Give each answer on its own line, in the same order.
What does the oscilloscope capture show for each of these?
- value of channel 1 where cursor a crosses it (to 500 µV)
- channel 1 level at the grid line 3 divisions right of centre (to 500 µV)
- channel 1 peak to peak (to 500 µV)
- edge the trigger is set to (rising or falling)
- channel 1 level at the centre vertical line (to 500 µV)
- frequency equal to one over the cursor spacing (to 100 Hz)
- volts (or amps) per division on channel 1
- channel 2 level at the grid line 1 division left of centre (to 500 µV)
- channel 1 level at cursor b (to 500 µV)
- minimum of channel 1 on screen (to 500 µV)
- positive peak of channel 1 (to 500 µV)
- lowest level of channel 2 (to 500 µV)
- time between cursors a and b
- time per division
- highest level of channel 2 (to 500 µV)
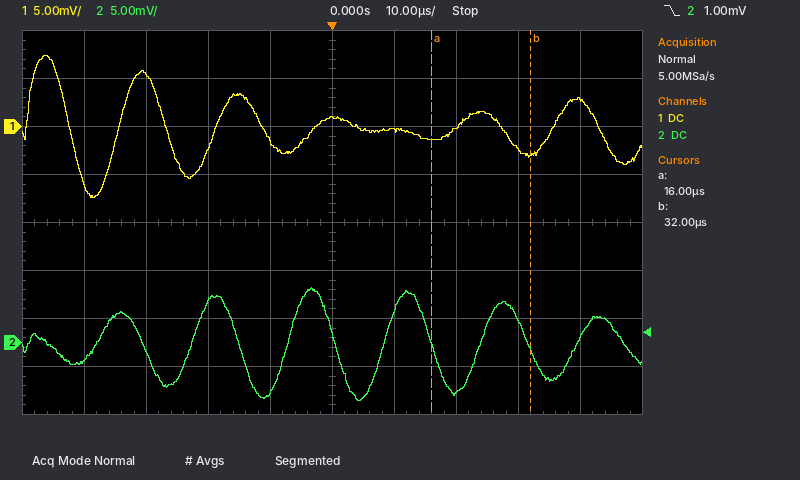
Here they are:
-1.5 mV
-2.5 mV
15.0 mV
falling
1.0 mV
62.5 kHz
5 mV
-5.0 mV
-3.0 mV
-7.5 mV
7.5 mV
-6.0 mV
16 µs
10 µs
5.5 mV
